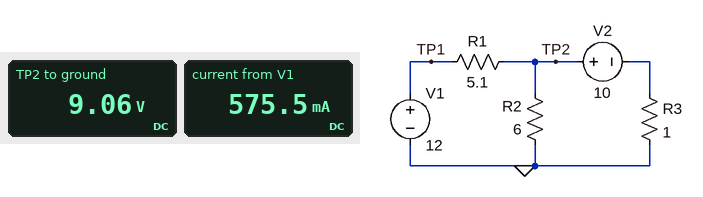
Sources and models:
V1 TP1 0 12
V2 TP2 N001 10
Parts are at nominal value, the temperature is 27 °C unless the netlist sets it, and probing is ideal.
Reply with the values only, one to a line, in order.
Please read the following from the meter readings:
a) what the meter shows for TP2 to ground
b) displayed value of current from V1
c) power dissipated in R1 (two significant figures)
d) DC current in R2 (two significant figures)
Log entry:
9.06 V
575.5 mA
1.7 W
1.5 A
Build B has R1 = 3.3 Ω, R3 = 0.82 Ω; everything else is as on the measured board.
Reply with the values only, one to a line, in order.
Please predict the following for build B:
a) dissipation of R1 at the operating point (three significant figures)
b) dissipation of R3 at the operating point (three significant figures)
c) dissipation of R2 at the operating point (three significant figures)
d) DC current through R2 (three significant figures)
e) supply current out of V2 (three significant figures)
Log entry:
2.09 W
481 mW
14.6 W
1.56 A
766 mA
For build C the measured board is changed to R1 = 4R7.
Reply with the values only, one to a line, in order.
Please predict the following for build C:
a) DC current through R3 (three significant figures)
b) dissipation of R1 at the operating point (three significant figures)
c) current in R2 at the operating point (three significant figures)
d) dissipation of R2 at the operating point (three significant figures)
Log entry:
900 mA
1.79 W
1.52 A
13.8 W
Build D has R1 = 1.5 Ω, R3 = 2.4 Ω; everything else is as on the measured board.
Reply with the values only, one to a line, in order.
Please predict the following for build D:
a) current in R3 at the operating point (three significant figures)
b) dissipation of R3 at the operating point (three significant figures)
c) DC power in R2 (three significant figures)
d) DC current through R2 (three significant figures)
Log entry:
111 mA
29.6 mW
15.8 W
1.62 A
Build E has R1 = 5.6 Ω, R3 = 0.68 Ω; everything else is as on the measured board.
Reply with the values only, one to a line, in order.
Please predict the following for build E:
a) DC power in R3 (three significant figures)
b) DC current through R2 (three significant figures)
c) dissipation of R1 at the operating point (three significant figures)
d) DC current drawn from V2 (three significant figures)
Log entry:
765 mW
1.55 A
1.32 W
1.06 A
